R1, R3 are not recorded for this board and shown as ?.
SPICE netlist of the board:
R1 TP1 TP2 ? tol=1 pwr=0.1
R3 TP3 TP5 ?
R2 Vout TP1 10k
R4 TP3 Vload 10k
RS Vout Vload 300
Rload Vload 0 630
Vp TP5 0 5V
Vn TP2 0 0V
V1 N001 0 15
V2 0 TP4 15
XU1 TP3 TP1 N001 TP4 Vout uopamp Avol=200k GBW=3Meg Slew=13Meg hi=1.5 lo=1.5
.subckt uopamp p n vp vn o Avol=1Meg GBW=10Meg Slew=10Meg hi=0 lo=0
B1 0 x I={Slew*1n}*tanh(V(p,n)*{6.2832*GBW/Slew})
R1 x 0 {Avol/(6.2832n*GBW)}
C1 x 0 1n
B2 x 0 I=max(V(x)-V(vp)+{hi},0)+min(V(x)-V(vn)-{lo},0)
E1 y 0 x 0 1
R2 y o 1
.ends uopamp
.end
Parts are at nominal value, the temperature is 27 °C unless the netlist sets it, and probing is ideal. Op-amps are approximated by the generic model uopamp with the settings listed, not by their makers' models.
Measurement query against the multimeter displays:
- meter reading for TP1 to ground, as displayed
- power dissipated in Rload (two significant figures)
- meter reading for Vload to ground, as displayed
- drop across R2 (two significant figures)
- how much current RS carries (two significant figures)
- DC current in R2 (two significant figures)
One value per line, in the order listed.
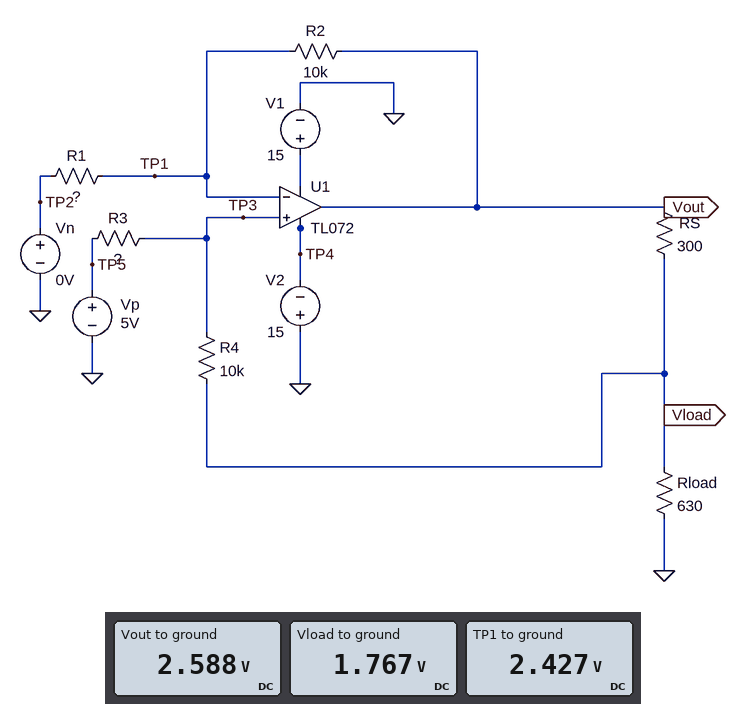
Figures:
2.427 V
5.0 mW
1.767 V
160 mV
2.7 mA
16 µA
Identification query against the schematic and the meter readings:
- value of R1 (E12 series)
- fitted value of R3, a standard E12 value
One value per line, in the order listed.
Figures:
150 kΩ
39 kΩ
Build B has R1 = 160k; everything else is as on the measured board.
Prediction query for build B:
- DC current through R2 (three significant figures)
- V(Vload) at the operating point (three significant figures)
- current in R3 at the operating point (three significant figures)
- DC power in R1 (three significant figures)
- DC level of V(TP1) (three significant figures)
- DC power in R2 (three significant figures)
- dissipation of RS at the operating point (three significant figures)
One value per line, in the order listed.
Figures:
15.1 µA
1.75 V
66.3 µA
36.4 µW
2.41 V
2.28 µW
2.21 mW
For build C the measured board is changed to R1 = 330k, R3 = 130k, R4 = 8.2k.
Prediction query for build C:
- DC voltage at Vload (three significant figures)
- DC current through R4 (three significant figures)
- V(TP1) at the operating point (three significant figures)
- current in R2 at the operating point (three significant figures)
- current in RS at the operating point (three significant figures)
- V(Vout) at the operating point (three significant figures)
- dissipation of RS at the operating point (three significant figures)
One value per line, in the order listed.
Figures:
622 mV
31.7 µA
881 mV
2.67 µA
955 µA
908 mV
274 µW
